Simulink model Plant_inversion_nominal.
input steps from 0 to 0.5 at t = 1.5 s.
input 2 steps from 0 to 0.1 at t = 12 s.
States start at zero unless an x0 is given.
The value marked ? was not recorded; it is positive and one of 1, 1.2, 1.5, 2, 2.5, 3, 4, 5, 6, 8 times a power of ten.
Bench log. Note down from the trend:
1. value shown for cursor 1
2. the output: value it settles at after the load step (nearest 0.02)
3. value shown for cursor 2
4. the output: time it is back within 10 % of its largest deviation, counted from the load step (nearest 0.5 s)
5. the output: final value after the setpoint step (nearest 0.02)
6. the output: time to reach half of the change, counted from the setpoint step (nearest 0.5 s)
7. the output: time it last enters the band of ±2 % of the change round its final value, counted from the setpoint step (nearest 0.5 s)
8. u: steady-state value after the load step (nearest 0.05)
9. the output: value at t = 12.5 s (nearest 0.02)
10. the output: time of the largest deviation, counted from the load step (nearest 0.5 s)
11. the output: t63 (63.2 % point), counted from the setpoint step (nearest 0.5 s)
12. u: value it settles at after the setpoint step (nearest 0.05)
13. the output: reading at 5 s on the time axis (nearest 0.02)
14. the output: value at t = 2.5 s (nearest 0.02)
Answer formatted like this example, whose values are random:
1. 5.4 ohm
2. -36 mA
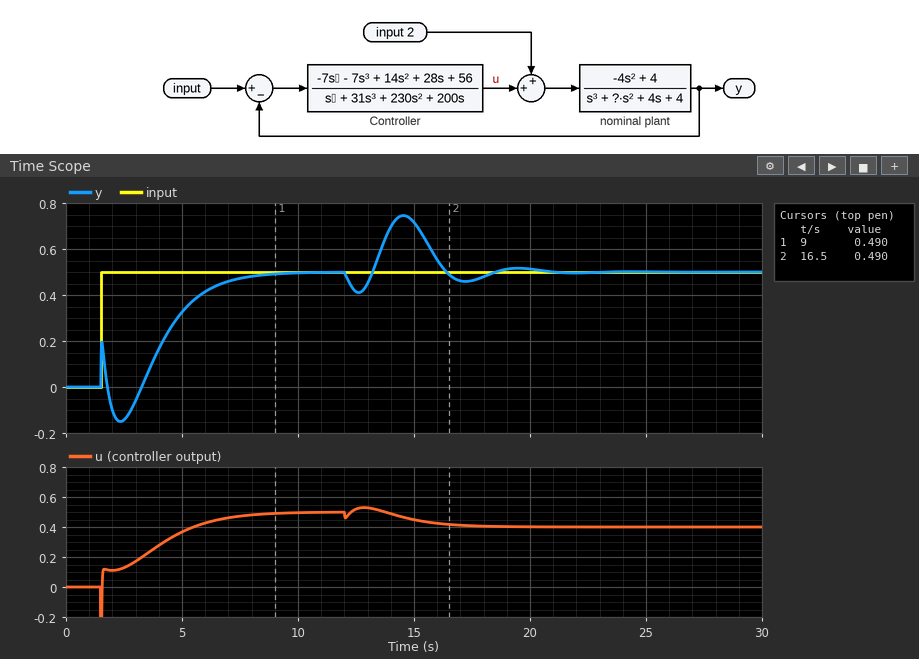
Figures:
1. 0.490
2. 0.50
3. 0.490
4. 6.0 s
5. 0.50
6. 3.0 s
7. 7.5 s
8. 0.40
9. 0.42
10. 2.5 s
11. 3.5 s
12. 0.50
13. 0.32
14. -0.14
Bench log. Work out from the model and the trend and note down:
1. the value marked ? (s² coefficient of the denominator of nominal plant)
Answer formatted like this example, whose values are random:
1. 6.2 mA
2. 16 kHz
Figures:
1. 3
